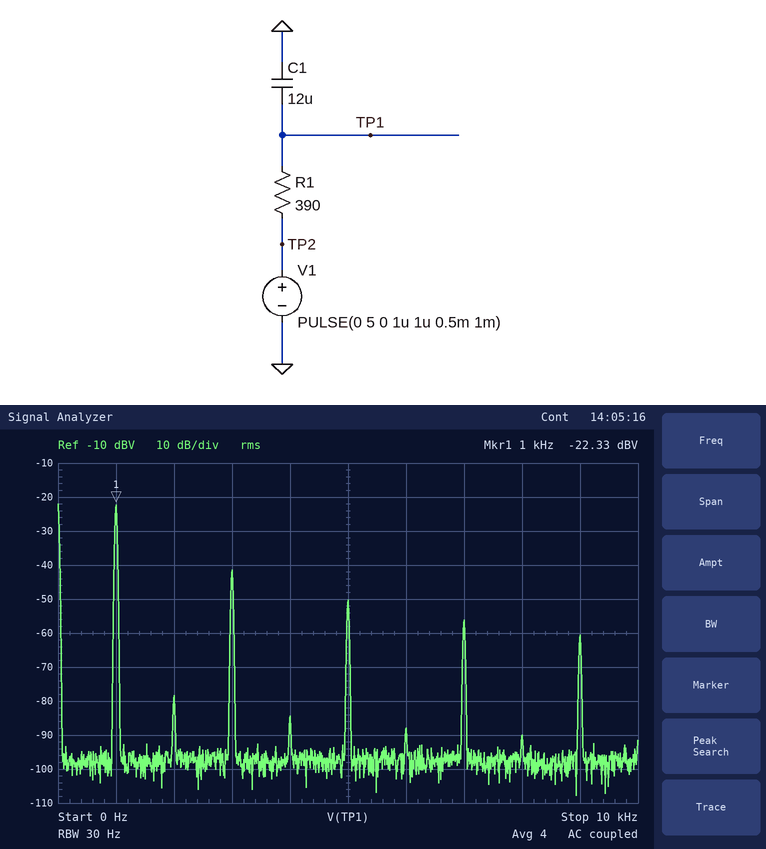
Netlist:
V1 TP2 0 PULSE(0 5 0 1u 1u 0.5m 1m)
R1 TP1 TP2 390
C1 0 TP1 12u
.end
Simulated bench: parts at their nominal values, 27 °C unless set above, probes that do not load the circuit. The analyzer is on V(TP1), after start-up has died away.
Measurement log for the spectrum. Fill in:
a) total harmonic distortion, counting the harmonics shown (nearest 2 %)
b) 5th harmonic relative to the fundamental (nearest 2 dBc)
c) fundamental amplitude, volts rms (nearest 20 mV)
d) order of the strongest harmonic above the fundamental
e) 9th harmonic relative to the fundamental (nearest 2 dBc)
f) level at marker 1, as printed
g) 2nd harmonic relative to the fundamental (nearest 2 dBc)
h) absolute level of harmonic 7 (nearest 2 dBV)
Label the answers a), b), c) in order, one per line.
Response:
a) 12 %
b) -28 dBc
c) 80 mV
d) 3
e) -38 dBc
f) -22.33 dBV
g) -56 dBc
h) -56 dBV
